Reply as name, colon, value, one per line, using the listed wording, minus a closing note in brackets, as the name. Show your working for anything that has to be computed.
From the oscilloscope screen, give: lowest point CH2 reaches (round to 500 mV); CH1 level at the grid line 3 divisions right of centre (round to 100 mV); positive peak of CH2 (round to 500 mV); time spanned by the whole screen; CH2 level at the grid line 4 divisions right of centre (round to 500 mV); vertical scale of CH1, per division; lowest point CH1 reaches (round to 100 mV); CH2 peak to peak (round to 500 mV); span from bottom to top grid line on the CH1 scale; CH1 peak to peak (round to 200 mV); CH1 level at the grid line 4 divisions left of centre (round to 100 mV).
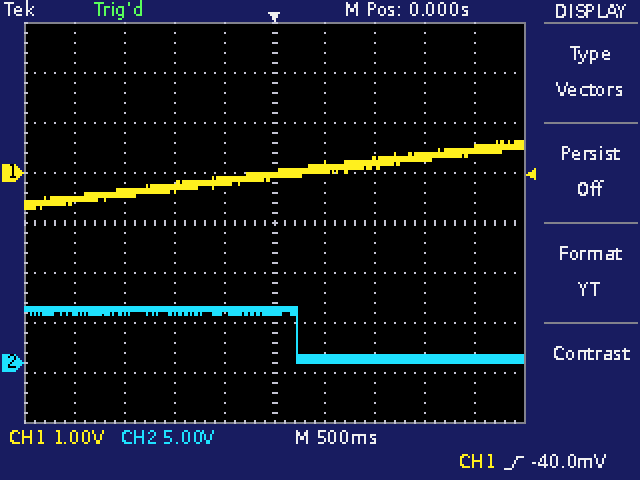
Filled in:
lowest point CH2 reaches: 0.0 V
CH1 level at the grid line 3 divisions right of centre: 300 mV
positive peak of CH2: 5.5 V
time spanned by the whole screen: 5 s
CH2 level at the grid line 4 divisions right of centre: 500 mV
vertical scale of CH1, per division: 1 V
lowest point CH1 reaches: -700 mV
CH2 peak to peak: 5.5 V − (0.0 V) = 5.5 V
span from bottom to top grid line on the CH1 scale: 8 V
CH1 peak to peak: 1.4 V
CH1 level at the grid line 4 divisions left of centre: -600 mV
